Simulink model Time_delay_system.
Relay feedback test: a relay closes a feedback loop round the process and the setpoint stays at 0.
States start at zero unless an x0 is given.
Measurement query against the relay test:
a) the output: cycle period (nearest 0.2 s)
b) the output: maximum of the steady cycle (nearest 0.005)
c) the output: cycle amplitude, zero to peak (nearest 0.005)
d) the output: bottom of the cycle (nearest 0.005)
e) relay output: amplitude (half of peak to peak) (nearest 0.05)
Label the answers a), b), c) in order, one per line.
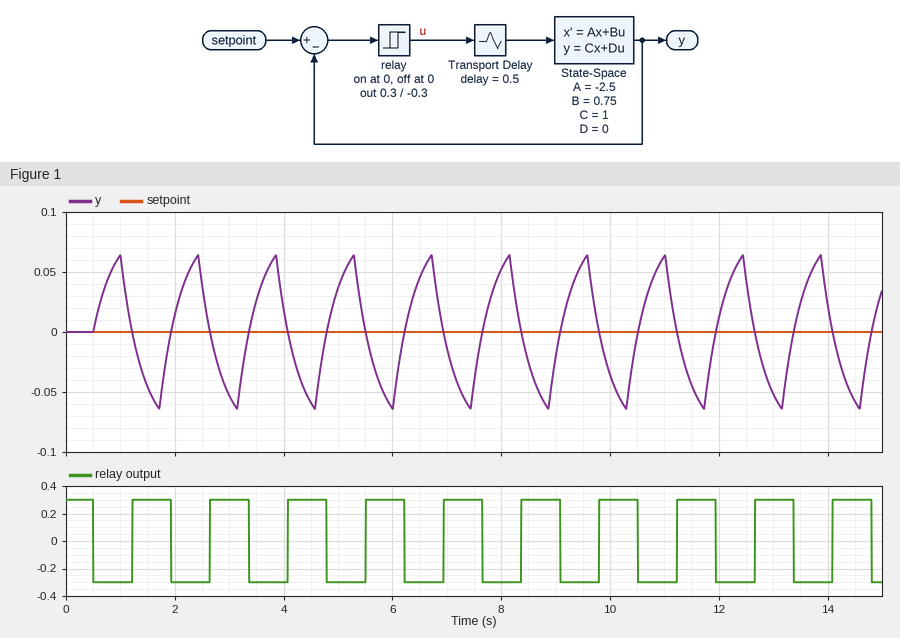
a) 1.4 s
b) 0.065
c) 0.065
d) -0.065
e) 0.30
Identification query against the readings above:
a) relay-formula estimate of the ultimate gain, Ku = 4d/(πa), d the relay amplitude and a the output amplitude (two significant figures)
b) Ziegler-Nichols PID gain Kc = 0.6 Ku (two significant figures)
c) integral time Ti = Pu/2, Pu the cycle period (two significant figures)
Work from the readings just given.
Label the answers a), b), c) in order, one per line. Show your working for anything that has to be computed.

a) 4 × 0.3 / (π × 0.065) = 5.9
b) 0.6 × 5.9 = 3.5
c) 1.4 / 2 = 0.70 s
